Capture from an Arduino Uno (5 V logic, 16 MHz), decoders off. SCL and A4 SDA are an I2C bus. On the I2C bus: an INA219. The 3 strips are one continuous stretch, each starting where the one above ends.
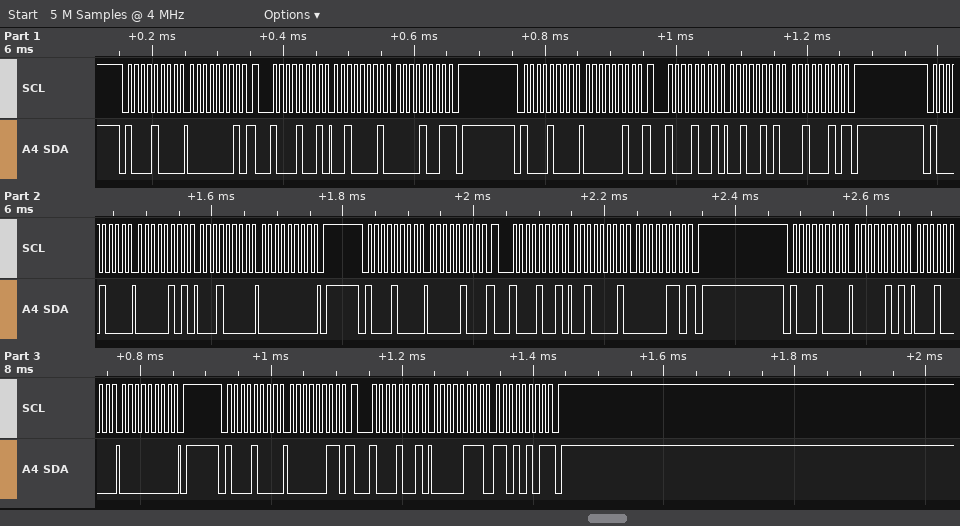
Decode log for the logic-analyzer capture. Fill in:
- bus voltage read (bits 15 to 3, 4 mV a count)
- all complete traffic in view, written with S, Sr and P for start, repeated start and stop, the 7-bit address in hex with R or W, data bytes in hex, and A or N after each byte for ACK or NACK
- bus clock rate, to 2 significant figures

4.752 V
S 44W A 01 A Sr 44R A 21 A 09 N P S 44W A 02 A Sr 44R A 25 A 22 N P S 44W A 05 A 10 A 00 A P S 44W A 04 A Sr 44R A 21 A 06 N P S 44W A 05 A 10 A 00 A P S 44W A 03 A Sr 44R A 07 A D5 N P
100 kHz
